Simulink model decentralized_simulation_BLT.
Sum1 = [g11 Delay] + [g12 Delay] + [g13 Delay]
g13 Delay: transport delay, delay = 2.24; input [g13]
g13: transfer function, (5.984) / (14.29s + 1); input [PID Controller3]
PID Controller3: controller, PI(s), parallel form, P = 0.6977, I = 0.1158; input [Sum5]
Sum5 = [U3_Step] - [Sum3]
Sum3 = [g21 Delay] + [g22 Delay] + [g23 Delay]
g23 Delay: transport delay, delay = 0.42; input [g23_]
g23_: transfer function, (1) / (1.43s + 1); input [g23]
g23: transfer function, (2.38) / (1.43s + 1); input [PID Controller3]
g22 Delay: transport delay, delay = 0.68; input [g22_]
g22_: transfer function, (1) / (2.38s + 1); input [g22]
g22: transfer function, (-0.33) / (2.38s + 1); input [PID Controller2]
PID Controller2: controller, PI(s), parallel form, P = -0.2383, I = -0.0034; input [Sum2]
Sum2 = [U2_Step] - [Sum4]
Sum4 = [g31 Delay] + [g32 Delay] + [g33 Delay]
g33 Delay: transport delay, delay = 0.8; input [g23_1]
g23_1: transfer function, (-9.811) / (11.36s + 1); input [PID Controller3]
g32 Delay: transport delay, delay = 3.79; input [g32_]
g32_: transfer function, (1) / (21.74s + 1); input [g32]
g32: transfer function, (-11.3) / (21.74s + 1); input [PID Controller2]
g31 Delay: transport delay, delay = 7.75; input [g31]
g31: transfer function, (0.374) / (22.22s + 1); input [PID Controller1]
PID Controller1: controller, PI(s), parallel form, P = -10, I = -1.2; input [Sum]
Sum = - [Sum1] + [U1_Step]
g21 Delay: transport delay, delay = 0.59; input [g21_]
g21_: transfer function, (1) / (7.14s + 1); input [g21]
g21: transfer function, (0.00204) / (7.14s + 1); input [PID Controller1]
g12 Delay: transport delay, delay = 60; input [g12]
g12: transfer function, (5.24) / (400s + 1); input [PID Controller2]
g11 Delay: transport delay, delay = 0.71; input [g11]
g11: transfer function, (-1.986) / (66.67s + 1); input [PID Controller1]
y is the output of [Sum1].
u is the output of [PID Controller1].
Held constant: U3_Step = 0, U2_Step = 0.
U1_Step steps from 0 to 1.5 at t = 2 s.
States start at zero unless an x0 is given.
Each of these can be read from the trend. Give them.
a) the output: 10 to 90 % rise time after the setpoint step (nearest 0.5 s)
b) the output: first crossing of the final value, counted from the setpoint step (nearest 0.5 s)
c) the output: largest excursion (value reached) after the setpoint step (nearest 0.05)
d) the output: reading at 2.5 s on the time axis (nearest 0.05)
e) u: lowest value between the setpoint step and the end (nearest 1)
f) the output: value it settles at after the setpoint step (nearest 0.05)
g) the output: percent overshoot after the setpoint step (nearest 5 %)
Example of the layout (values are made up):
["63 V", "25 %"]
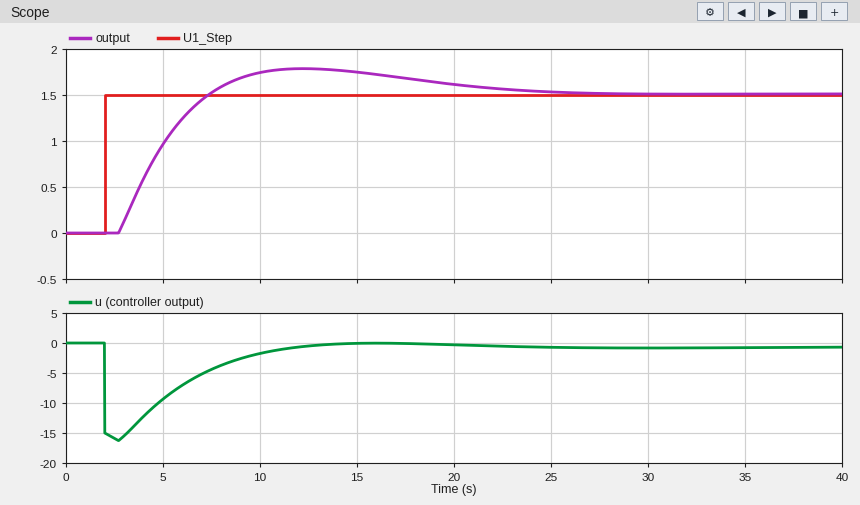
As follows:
["3.5 s", "5.5 s", "1.80", "0.00", "-16", "1.50", "20 %"]
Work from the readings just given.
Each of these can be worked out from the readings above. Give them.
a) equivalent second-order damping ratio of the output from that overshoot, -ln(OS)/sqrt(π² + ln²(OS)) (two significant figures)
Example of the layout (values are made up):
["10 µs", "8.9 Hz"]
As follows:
["0.46"]
